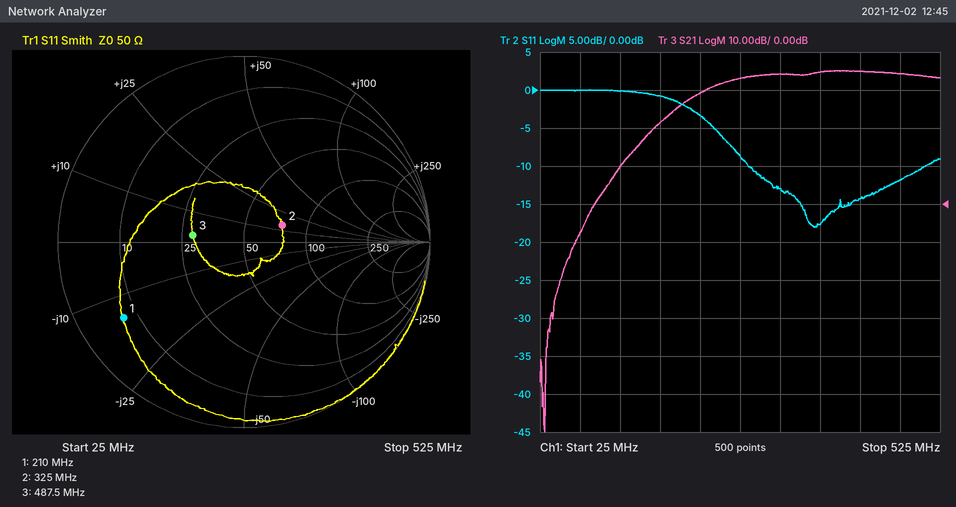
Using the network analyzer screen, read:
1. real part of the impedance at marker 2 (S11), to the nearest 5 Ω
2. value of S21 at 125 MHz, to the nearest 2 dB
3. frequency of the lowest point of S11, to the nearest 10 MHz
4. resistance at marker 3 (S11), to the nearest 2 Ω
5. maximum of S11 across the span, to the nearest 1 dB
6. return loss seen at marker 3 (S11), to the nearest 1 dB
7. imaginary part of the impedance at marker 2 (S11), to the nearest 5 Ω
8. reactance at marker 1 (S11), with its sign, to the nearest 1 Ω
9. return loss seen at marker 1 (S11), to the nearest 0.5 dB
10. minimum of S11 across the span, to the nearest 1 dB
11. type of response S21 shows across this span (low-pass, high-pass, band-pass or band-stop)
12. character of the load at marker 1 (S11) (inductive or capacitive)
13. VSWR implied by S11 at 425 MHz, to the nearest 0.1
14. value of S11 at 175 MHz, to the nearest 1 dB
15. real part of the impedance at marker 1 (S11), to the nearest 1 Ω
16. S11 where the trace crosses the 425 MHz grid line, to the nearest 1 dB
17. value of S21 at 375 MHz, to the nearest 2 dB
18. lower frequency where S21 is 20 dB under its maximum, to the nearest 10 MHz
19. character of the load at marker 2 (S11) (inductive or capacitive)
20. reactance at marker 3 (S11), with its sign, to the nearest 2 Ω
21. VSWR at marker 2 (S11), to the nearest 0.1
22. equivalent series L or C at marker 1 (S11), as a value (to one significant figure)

75 Ω
10 dB
370 MHz
28 Ω
0 dB
11 dB
+15 Ω
-14 Ω
2.5 dB
-18 dB
high-pass
capacitive
1.5
-1 dB
7 Ω
-14 dB
34 dB
150 MHz
inductive
+2 Ω
1.6
50 pF
